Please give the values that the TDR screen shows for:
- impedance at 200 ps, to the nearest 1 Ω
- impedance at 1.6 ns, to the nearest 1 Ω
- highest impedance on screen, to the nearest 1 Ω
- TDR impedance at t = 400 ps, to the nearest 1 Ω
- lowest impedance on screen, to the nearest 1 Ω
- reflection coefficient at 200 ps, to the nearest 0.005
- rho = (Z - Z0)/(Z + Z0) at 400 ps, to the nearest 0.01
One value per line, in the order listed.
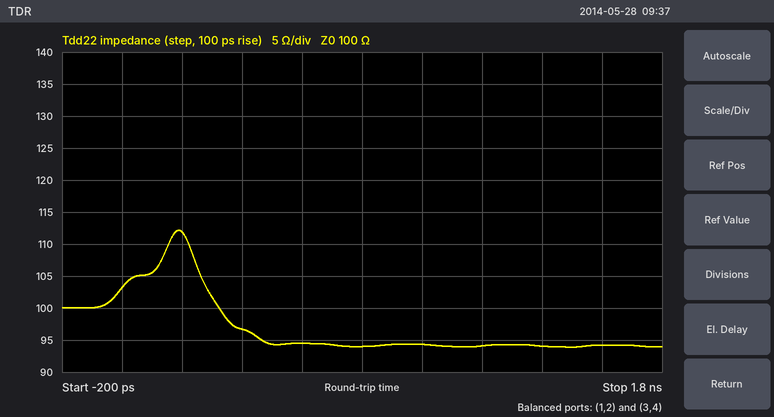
112 Ω
94 Ω
112 Ω
97 Ω
94 Ω
+0.055
-0.02
